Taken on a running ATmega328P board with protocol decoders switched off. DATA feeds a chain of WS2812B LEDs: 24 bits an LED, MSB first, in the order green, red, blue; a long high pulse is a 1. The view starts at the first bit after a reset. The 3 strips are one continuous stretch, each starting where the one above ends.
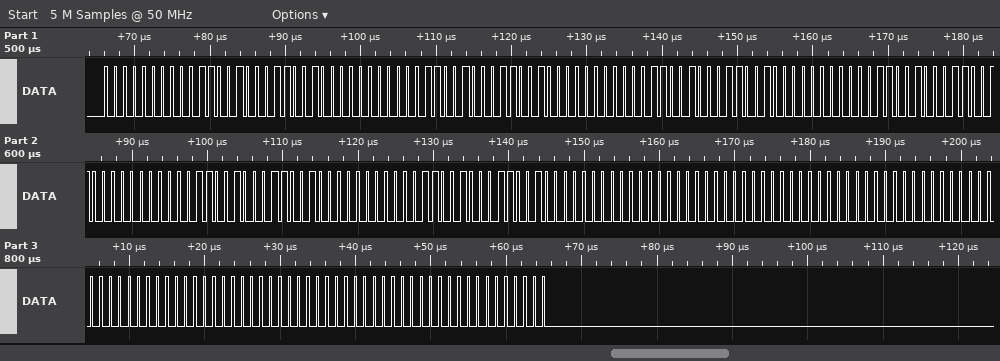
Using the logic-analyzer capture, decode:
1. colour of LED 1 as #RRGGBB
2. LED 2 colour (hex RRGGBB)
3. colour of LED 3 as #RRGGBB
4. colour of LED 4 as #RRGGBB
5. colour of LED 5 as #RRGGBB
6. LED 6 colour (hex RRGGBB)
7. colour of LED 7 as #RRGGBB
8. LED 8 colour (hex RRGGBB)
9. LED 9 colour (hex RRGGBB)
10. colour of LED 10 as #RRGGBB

#320032
#320032
#320032
#320032
#320032
#320032
#000000
#000000
#000000
#000000
